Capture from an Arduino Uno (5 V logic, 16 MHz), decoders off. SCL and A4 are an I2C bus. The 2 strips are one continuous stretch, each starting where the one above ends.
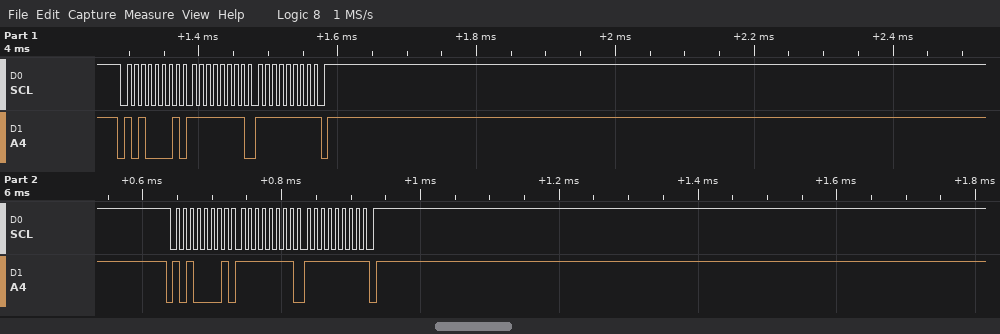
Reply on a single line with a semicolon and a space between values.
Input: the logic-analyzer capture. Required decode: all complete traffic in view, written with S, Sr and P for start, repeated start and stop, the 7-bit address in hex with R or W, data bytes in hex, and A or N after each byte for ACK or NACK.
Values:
S 50R A FF A FF N P S 50R A FF A FF N P
